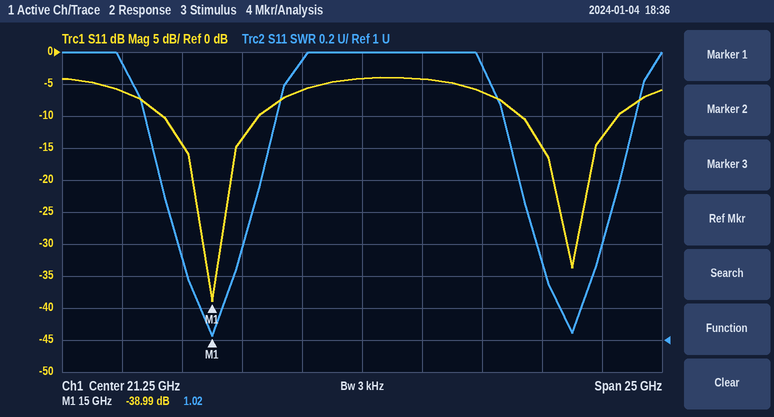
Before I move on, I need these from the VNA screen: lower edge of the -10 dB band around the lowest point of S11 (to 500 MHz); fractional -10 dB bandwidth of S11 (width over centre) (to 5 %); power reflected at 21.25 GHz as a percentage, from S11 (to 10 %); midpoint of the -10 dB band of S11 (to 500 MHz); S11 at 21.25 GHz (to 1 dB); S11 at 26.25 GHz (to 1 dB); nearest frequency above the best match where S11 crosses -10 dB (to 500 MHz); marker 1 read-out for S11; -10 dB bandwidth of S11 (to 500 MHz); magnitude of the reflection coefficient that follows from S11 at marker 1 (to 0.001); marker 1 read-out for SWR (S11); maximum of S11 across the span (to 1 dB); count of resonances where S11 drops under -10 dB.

13.0 GHz
25 %
40 %
15.0 GHz
-4 dB
-6 dB
17.0 GHz
-38.99 dB
4.0 GHz
0.011
1.02
-4 dB
2
